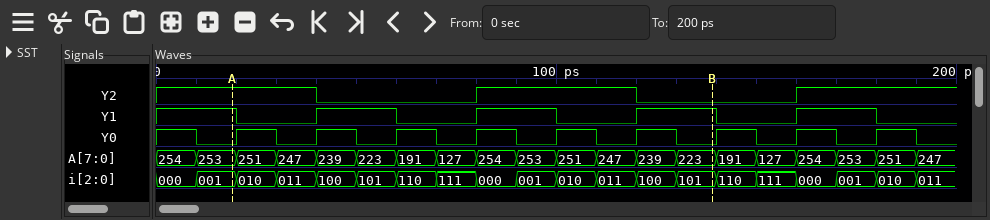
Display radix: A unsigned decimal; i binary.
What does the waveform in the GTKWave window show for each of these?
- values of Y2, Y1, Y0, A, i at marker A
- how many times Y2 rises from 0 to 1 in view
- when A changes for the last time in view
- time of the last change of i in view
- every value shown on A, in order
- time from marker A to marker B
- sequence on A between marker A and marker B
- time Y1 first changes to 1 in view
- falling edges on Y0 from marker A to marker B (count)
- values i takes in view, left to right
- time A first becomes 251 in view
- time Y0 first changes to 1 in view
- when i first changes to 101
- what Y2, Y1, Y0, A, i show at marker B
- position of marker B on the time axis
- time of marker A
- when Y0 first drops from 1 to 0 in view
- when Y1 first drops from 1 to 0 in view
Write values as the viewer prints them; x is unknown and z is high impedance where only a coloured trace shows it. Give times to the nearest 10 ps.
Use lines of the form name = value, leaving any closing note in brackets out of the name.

values of Y2, Y1, Y0, A, i at marker A = Y2=1, Y1=1, Y0=0, A=253, i=001
how many times Y2 rises from 0 to 1 in view = 2
when A changes for the last time in view = 190 ps
time of the last change of i in view = 190 ps
every value shown on A, in order = 254, 253, 251, 247, 239, 223, 191, 127, 254, 253, 251, 247, 239, 223, 191, 127, 254, 253, 251, 247
time from marker A to marker B = 120 ps
sequence on A between marker A and marker B = 253, 251, 247, 239, 223, 191, 127, 254, 253, 251, 247, 239, 223
time Y1 first changes to 1 in view = 40 ps
falling edges on Y0 from marker A to marker B = 6
values i takes in view, left to right = 000, 001, 010, 011, 100, 101, 110, 111, 000, 001, 010, 011, 100, 101, 110, 111, 000, 001, 010, 011
time A first becomes 251 in view = 20 ps
time Y0 first changes to 1 in view = 20 ps
when i first changes to 101 = 50 ps
what Y2, Y1, Y0, A, i show at marker B = Y2=0, Y1=1, Y0=0, A=223, i=101
position of marker B on the time axis = 140 ps
time of marker A = 20 ps
when Y0 first drops from 1 to 0 in view = 10 ps
when Y1 first drops from 1 to 0 in view = 20 ps
